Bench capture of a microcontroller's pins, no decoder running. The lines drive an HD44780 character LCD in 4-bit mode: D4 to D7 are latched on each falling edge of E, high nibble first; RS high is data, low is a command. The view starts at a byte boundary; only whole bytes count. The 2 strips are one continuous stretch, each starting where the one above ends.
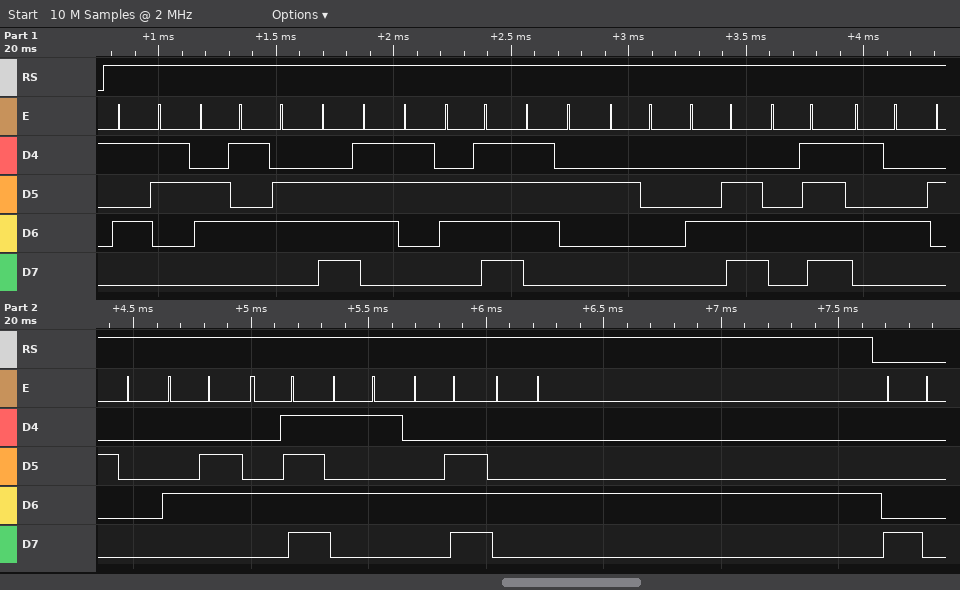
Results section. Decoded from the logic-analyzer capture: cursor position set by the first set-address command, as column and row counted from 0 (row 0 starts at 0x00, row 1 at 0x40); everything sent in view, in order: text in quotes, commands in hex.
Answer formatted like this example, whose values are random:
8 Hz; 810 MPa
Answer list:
column 0, row 0; "Sensor NOT FOUND" 0x80
